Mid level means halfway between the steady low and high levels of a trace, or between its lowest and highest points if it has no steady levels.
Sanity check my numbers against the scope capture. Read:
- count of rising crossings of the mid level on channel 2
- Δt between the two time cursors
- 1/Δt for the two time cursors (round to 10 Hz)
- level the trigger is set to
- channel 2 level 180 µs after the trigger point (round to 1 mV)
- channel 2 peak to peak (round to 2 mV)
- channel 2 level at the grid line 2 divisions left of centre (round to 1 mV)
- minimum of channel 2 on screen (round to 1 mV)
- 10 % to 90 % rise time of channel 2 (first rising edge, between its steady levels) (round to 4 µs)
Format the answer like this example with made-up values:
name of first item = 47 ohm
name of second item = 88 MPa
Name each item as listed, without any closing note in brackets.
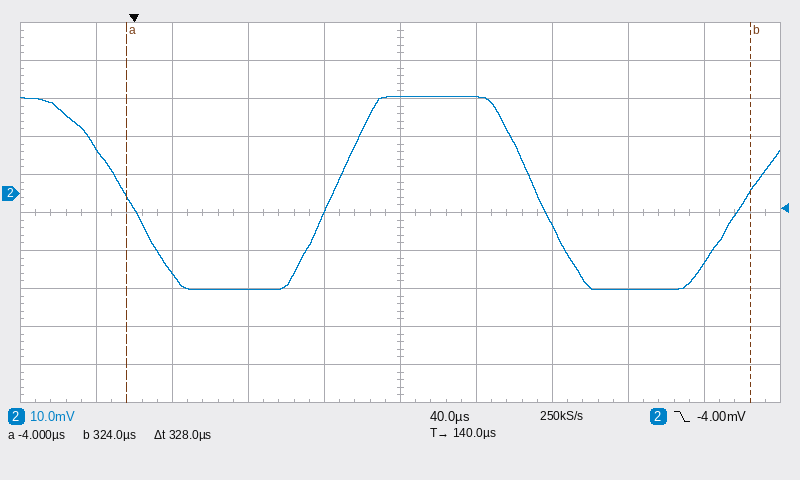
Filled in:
count of rising crossings of the mid level on channel 2 = 2
Δt between the two time cursors = 328 µs
1/Δt for the two time cursors = 3.05 kHz
level the trigger is set to = -4.00 mV
channel 2 level 180 µs after the trigger point = 25 mV
channel 2 peak to peak = 50 mV
channel 2 level at the grid line 2 divisions left of centre = -25 mV
minimum of channel 2 on screen = -25 mV
10 % to 90 % rise time of channel 2 (first rising edge, between its steady levels) = 40 µs
